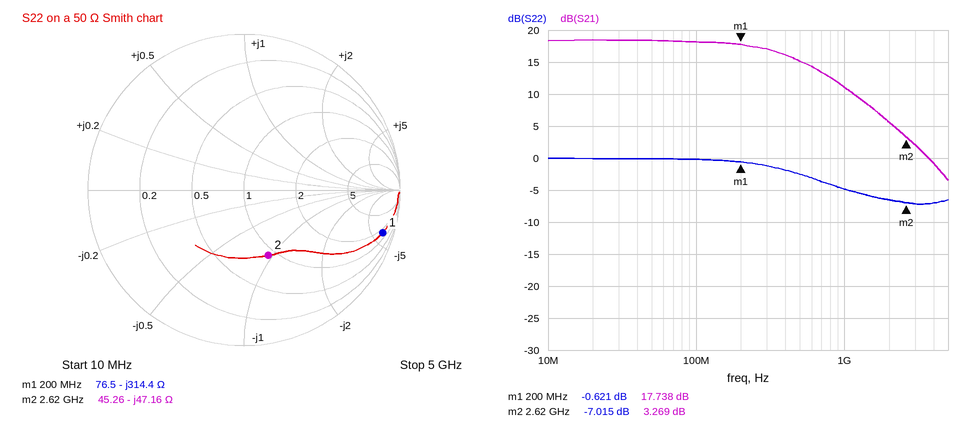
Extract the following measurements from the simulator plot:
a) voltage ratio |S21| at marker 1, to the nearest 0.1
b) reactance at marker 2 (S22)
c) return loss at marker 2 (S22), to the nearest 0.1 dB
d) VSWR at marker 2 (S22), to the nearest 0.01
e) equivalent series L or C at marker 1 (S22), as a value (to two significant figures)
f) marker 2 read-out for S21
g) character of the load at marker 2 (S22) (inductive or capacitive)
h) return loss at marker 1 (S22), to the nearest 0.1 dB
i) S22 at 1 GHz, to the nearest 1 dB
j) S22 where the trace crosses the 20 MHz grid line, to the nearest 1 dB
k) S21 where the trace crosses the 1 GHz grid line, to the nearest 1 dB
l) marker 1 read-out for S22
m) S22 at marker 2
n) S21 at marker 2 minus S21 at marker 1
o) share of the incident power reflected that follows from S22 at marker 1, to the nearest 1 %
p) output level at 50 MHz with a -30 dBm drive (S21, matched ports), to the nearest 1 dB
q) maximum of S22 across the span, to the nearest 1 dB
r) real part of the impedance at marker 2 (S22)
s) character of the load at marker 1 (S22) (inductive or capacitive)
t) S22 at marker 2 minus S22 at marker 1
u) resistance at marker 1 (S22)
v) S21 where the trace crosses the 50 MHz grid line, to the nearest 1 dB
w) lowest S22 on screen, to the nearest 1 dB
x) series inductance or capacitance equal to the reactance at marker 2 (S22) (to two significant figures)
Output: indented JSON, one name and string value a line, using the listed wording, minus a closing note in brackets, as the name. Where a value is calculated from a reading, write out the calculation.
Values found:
{
  "voltage ratio |S21| at marker 1, to the nearest 0.1": "10^(17.738/20) ≈ 7.7",
  "reactance at marker 2": "-47.16 Ω",
  "return loss at marker 2 (S22), to the nearest 0.1 dB": "7.0 dB",
  "VSWR at marker 2 (S22), to the nearest 0.01": "(1 + 0.4459)/(1 − 0.4459) ≈ 2.61",
  "equivalent series L or C at marker 1 (S22), as a value": "C = 1/(2π × 200 MHz × 314.4 Ω) ≈ 2.5 pF",
  "marker 2 read-out for S21": "3.269 dB",
  "character of the load at marker 2 (S22)": "capacitive",
  "return loss at marker 1 (S22), to the nearest 0.1 dB": "0.6 dB",
  "S22 at 1 GHz, to the nearest 1 dB": "-5 dB",
  "S22 where the trace crosses the 20 MHz grid line, to the nearest 1 dB": "0 dB",
  "S21 where the trace crosses the 1 GHz grid line, to the nearest 1 dB": "11 dB",
  "marker 1 read-out for S22": "-0.621 dB",
  "S22 at marker 2": "-7.015 dB",
  "S21 at marker 2 minus S21 at marker 1": "3.269 − (17.738) = -14.469 dB",
  "share of the incident power reflected that follows from S22 at marker 1, to the nearest 1 %": "10^(-0.621/10) ≈ 87 %",
  "output level at 50 MHz with a -30 dBm drive (S21, matched ports), to the nearest 1 dB": "-30 dBm + (18 dB) = -12 dBm",
  "maximum of S22 across the span, to the nearest 1 dB": "0 dB",
  "real part of the impedance at marker 2": "45.26 Ω",
  "character of the load at marker 1 (S22)": "capacitive",
  "S22 at marker 2 minus S22 at marker 1": "-7.015 − (-0.621) = -6.394 dB",
  "resistance at marker 1": "76.5 Ω",
  "S21 where the trace crosses the 50 MHz grid line, to the nearest 1 dB": "18 dB",
  "lowest S22 on screen, to the nearest 1 dB": "-7 dB",
  "series inductance or capacitance equal to the reactance at marker 2 (S22)": "C = 1/(2π × 2.62 GHz × 47.16 Ω) ≈ 1.3 pF"
}
